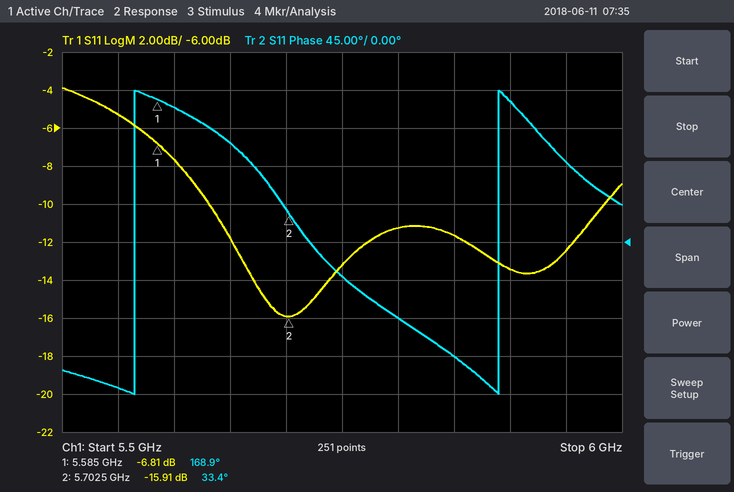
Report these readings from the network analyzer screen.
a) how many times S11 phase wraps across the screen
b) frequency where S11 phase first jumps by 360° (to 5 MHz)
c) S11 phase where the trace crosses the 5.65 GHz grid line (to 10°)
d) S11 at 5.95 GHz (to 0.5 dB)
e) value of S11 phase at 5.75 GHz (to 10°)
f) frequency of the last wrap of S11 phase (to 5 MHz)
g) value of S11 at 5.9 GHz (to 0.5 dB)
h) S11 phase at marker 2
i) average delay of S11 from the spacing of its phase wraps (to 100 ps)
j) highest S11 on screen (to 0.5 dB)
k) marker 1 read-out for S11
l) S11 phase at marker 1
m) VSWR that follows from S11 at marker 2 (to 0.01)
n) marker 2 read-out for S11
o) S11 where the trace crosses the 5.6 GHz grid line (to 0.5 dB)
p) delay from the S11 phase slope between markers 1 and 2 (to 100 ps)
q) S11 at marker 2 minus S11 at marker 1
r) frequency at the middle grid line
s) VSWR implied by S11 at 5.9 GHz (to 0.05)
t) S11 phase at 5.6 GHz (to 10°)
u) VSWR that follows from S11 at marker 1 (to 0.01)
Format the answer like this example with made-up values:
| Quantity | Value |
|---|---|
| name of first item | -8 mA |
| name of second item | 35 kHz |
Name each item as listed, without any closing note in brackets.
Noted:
| Quantity | Value |
|---|---|
| how many times S11 phase wraps across the screen | 2 |
| frequency where S11 phase first jumps by 360° | 5.565 GHz |
| S11 phase where the trace crosses the 5.65 GHz grid line | 120° |
| S11 at 5.95 GHz | -12.5 dB |
| value of S11 phase at 5.75 GHz | -40° |
| frequency of the last wrap of S11 phase | 5.890 GHz |
| value of S11 at 5.9 GHz | -13.5 dB |
| S11 phase at marker 2 | 33.4° |
| average delay of S11 from the spacing of its phase wraps | 3.1 ns |
| highest S11 on screen | -4.0 dB |
| marker 1 read-out for S11 | -6.81 dB |
| S11 phase at marker 1 | 168.9° |
| VSWR that follows from S11 at marker 2 | 1.38 |
| marker 2 read-out for S11 | -15.91 dB |
| S11 where the trace crosses the 5.6 GHz grid line | -7.5 dB |
| delay from the S11 phase slope between markers 1 and 2 | 3.2 ns |
| S11 at marker 2 minus S11 at marker 1 | -9.10 dB |
| frequency at the middle grid line | 5.75 GHz |
| VSWR implied by S11 at 5.9 GHz | 1.55 |
| S11 phase at 5.6 GHz | 160° |
| VSWR that follows from S11 at marker 1 | 2.68 |
